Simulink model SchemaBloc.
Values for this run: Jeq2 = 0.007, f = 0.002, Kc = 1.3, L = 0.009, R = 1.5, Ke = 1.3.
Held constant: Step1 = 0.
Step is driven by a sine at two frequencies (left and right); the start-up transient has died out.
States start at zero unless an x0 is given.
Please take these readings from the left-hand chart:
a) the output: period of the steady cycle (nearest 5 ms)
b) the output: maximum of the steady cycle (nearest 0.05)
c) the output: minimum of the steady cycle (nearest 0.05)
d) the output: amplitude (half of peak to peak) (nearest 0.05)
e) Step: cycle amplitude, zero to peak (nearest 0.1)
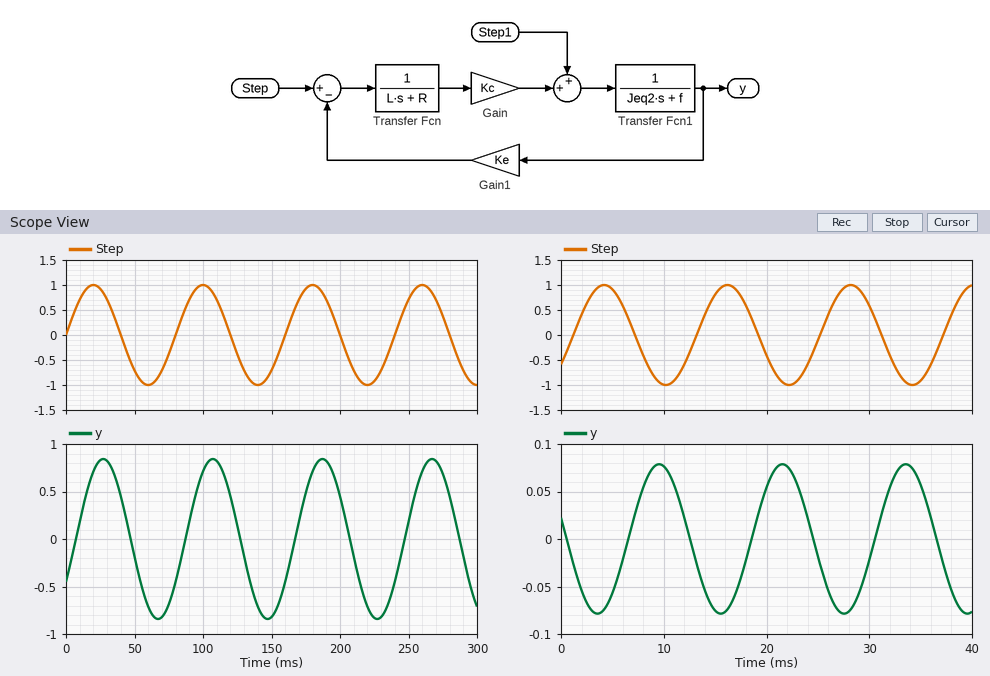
80 ms
0.85
-0.85
0.85
1.0
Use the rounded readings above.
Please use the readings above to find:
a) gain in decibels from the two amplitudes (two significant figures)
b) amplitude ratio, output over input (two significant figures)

-1.4 dB
0.85
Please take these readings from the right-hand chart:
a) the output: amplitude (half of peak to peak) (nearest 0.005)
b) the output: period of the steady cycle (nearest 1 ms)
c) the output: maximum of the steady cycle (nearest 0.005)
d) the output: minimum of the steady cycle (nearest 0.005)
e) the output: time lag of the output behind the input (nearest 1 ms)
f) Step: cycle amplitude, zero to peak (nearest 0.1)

0.080
12 ms
0.080
-0.080
5 ms
1.0
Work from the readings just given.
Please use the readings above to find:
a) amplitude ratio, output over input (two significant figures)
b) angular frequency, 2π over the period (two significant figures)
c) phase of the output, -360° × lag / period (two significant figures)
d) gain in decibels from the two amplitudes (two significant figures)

0.080
0.52 rad/ms
-150°
-22 dB
